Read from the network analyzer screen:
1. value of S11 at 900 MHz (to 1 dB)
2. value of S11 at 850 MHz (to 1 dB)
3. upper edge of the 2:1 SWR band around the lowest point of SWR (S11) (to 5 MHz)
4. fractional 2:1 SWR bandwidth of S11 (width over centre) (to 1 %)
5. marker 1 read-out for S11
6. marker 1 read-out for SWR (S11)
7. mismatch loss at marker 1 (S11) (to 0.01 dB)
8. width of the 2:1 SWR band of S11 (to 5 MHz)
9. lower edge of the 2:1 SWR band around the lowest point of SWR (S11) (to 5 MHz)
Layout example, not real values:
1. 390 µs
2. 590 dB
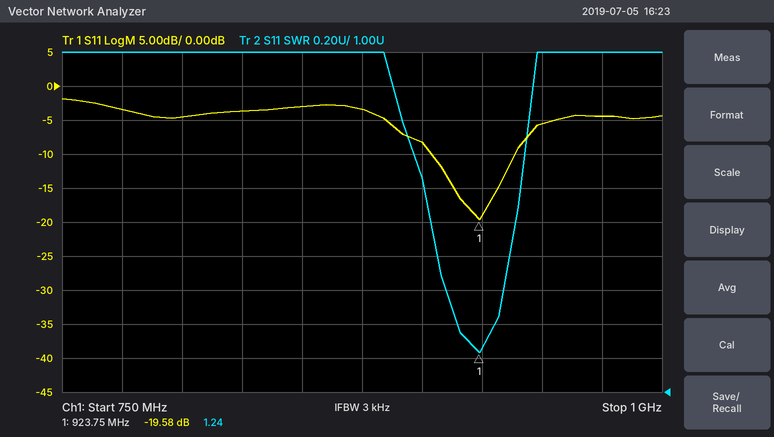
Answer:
1. -8 dB
2. -3 dB
3. 940 MHz
4. 4 %
5. -19.58 dB
6. 1.24
7. 0.05 dB
8. 35 MHz
9. 905 MHz
